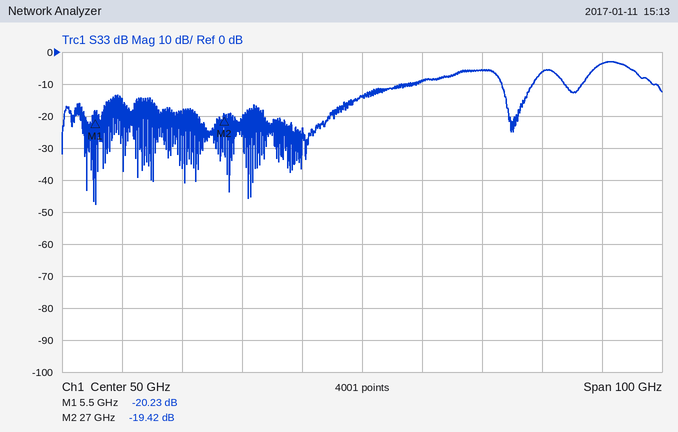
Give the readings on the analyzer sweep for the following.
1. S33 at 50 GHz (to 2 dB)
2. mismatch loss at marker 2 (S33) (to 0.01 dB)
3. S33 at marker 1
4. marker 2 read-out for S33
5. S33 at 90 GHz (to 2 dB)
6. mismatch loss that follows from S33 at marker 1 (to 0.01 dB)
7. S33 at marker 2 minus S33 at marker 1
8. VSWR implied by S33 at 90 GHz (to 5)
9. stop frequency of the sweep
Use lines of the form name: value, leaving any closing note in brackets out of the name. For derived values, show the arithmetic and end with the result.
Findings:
S33 at 50 GHz: -14 dB
mismatch loss at marker 2 (S33): −10 log10(1 − 10^(-19.42/10)) ≈ 0.05 dB
S33 at marker 1: -20.23 dB
marker 2 read-out for S33: -19.42 dB
S33 at 90 GHz: -4 dB
mismatch loss that follows from S33 at marker 1: −10 log10(1 − 10^(-20.23/10)) ≈ 0.04 dB
S33 at marker 2 minus S33 at marker 1: -19.42 − (-20.23) = 0.81 dB
VSWR implied by S33 at 90 GHz: |Γ| = 10^(-4/20) = 0.6310; VSWR = (1 + 0.6310)/(1 − 0.6310) ≈ 4.42, so 5 to the nearest 5
stop frequency of the sweep: 100 GHz
